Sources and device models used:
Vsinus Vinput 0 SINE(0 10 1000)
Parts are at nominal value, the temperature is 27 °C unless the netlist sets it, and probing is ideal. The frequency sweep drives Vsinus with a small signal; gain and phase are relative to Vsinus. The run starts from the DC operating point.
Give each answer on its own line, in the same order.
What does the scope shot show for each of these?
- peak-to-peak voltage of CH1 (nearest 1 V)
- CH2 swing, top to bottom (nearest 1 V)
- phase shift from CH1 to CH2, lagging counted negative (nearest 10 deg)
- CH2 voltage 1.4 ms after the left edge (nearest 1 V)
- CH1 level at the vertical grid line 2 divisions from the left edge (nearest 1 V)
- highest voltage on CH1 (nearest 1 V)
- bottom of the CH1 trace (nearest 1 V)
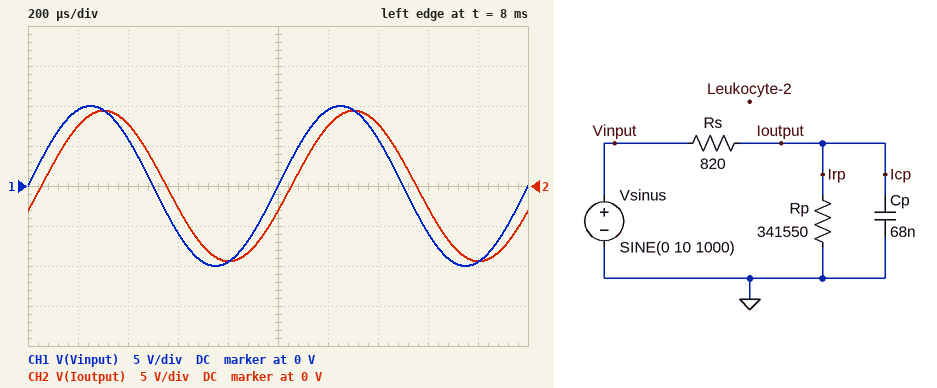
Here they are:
20 V
19 V
-20 deg
8 V
6 V
10 V
-10 V
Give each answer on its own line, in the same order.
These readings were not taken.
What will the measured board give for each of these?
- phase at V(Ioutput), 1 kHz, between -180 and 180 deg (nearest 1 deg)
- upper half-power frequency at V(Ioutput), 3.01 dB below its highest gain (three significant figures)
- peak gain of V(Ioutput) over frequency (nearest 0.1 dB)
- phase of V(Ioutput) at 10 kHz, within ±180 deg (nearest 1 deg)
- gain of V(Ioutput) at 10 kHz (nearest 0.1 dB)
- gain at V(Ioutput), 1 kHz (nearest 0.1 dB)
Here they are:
-19 deg
2.86 kHz
0 dB
-74 deg
-11.2 dB
-0.5 dB
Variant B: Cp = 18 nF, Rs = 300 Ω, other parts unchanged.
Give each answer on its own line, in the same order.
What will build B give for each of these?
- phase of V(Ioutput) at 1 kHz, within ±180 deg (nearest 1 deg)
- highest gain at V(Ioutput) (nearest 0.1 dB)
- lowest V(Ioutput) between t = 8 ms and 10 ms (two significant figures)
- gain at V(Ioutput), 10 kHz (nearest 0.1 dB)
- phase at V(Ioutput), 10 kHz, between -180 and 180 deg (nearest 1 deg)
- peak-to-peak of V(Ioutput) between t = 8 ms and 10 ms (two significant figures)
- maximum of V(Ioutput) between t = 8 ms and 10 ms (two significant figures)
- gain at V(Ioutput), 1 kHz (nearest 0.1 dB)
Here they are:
-2 deg
0 dB
-10 V
-0.5 dB
-19 deg
20 V
10 V
0 dB
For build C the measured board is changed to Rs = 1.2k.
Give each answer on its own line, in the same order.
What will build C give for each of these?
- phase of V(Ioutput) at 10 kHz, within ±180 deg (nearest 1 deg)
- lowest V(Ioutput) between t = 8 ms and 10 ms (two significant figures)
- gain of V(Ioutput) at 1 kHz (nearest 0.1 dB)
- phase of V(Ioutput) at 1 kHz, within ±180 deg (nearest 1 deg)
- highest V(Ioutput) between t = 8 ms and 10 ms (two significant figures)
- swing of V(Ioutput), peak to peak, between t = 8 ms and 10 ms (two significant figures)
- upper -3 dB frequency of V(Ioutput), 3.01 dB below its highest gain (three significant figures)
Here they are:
-79 deg
-8.9 V
-1.0 dB
-27 deg
8.9 V
18 V
1.96 kHz
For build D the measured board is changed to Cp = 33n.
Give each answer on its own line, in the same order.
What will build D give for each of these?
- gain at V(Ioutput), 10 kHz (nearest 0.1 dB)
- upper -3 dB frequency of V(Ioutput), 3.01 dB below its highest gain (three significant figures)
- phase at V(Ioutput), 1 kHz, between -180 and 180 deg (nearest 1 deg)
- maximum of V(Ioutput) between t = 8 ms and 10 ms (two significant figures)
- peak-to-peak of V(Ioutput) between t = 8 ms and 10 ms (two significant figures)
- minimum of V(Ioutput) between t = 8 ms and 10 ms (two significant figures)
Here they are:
-5.9 dB
5.90 kHz
-10 deg
9.8 V
20 V
-9.8 V
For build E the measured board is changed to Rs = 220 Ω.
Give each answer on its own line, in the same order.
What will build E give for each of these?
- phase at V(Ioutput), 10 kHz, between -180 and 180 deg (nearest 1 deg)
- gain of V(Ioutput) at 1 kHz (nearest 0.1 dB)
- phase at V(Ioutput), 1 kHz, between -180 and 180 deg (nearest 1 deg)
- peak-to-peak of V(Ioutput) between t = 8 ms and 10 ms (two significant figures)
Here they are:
-43 deg
0 dB
-5 deg
20 V
